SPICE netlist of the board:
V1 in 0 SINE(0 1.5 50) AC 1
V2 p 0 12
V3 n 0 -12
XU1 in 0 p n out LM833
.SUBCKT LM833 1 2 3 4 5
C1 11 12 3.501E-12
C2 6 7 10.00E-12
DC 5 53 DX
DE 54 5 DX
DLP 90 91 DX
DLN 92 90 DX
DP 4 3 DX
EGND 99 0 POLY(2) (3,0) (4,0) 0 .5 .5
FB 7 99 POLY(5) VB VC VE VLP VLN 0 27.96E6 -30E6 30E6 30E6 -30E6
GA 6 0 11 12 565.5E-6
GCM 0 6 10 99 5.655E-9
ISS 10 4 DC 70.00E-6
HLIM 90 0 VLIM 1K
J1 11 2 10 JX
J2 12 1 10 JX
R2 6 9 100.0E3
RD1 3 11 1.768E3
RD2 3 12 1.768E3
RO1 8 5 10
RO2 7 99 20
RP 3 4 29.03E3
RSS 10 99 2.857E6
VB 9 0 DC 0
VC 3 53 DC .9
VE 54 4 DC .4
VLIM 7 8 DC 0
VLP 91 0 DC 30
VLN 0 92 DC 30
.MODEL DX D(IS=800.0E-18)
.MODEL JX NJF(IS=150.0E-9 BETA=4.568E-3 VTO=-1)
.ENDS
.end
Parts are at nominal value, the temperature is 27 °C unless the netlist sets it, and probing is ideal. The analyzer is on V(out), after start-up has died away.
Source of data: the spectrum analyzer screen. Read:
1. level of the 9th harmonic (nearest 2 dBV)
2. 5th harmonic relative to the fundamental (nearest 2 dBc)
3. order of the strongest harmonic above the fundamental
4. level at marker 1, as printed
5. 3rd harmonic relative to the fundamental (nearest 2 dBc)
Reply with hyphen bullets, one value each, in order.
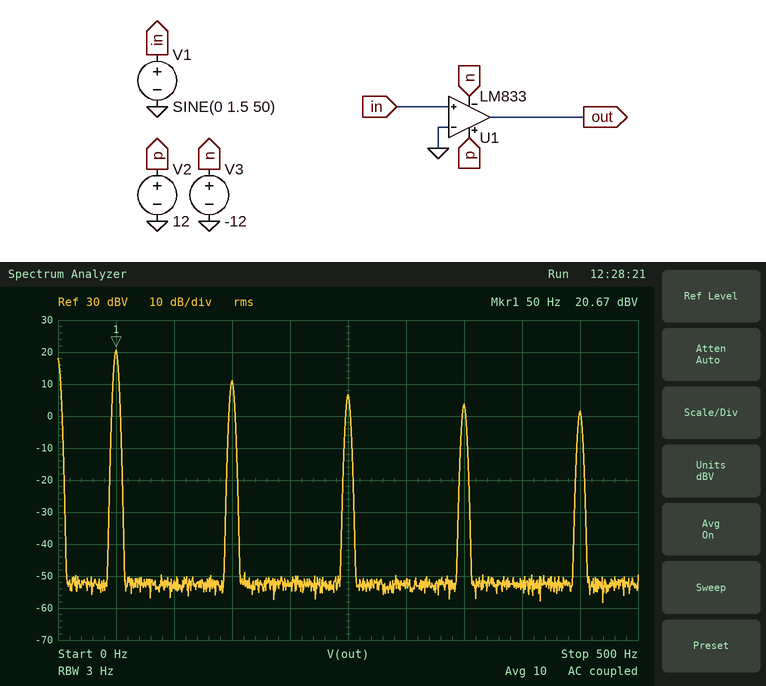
- 2 dBV
- -14 dBc
- 3
- 20.67 dBV
- -10 dBc
